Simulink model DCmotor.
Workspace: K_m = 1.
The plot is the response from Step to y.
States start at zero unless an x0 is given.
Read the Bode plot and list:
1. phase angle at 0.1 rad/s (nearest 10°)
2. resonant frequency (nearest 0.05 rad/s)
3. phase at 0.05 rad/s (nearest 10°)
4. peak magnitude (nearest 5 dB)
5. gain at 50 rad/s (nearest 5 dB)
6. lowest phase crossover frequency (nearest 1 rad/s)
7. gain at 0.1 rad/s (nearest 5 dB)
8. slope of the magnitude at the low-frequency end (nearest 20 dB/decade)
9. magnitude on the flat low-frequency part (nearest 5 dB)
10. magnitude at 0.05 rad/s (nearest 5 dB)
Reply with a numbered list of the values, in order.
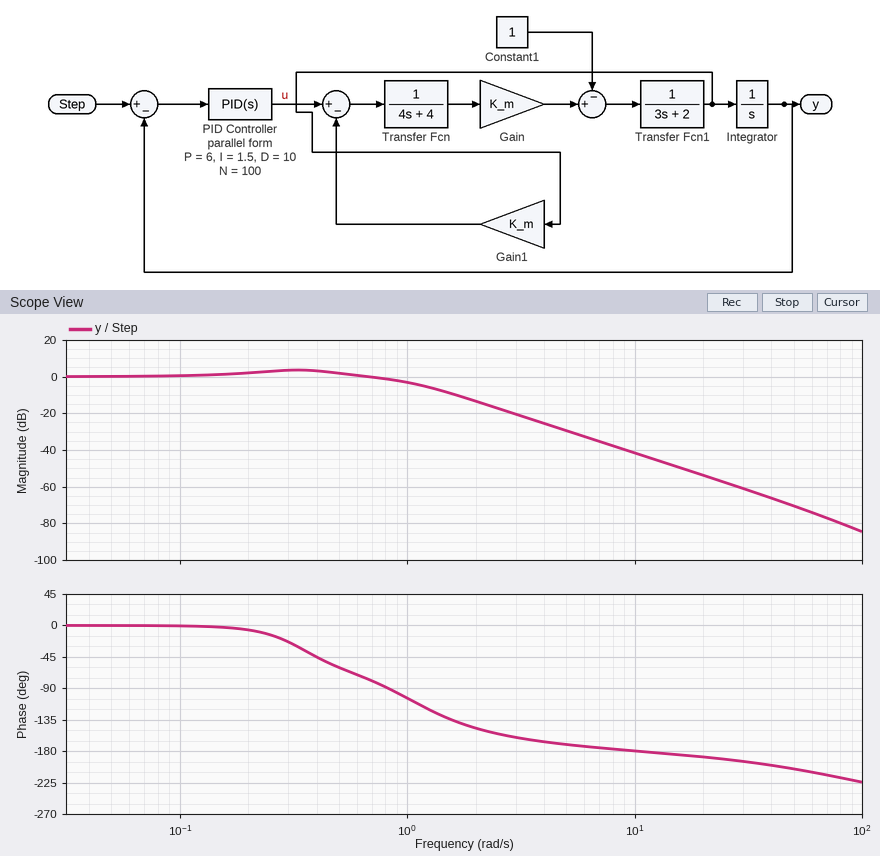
1. 0°
2. 0.35 rad/s
3. 0°
4. 5 dB
5. -70 dB
6. 10 rad/s
7. 0 dB
8. 0 dB/decade
9. 0 dB
10. 0 dB
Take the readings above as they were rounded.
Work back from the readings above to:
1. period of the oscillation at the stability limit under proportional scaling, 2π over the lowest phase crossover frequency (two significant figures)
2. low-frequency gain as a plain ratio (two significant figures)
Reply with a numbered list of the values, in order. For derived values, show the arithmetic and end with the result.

1. 2π / 10 = 0.63 s
2. 10^(0 / 20) = 1.0
